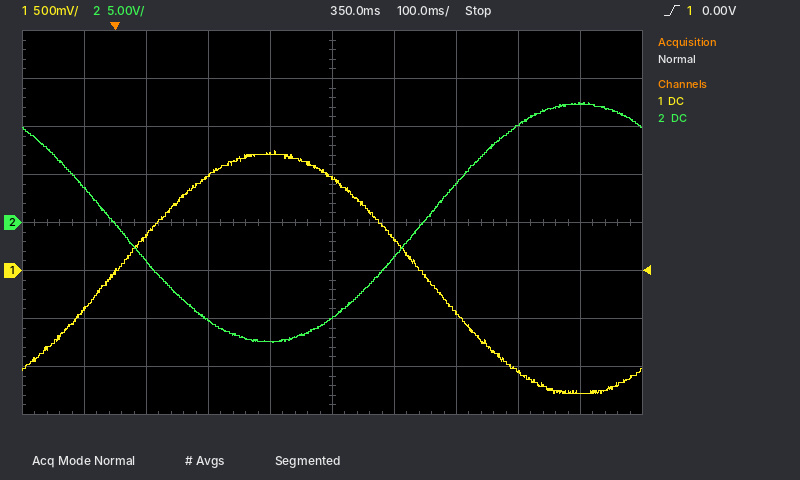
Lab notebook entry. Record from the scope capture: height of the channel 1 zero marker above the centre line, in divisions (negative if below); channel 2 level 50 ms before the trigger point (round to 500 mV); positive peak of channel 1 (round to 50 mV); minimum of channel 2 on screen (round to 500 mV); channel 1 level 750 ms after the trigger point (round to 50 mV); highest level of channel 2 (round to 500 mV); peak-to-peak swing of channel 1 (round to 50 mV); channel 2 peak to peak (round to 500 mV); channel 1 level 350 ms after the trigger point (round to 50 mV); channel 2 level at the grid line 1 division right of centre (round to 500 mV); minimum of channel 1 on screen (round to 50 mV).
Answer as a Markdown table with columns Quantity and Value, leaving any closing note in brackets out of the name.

| Quantity | Value |
|---|---|
| height of the channel 1 zero marker above the centre line, in divisions | -1.0 div |
| channel 2 level 50 ms before the trigger point | 3.5 V |
| positive peak of channel 1 | 1.25 V |
| minimum of channel 2 on screen | -12.5 V |
| channel 1 level 750 ms after the trigger point | -1.30 V |
| highest level of channel 2 | 12.5 V |
| peak-to-peak swing of channel 1 | 2.55 V |
| channel 2 peak to peak | 25.0 V |
| channel 1 level 350 ms after the trigger point | 950 mV |
| channel 2 level at the grid line 1 division right of centre | -3.5 V |
| minimum of channel 1 on screen | -1.30 V |
